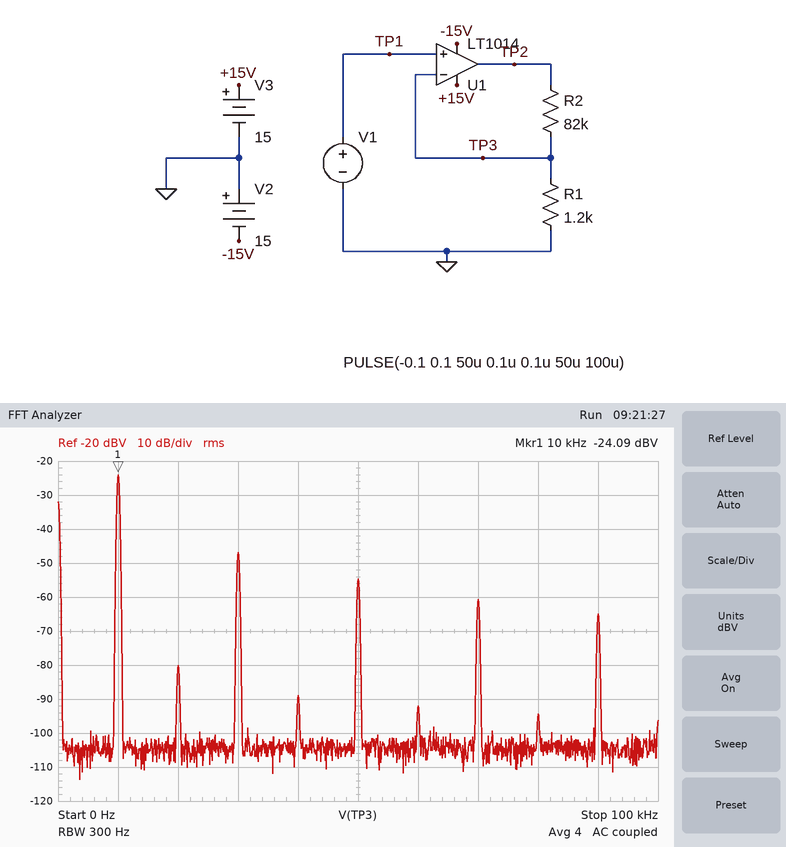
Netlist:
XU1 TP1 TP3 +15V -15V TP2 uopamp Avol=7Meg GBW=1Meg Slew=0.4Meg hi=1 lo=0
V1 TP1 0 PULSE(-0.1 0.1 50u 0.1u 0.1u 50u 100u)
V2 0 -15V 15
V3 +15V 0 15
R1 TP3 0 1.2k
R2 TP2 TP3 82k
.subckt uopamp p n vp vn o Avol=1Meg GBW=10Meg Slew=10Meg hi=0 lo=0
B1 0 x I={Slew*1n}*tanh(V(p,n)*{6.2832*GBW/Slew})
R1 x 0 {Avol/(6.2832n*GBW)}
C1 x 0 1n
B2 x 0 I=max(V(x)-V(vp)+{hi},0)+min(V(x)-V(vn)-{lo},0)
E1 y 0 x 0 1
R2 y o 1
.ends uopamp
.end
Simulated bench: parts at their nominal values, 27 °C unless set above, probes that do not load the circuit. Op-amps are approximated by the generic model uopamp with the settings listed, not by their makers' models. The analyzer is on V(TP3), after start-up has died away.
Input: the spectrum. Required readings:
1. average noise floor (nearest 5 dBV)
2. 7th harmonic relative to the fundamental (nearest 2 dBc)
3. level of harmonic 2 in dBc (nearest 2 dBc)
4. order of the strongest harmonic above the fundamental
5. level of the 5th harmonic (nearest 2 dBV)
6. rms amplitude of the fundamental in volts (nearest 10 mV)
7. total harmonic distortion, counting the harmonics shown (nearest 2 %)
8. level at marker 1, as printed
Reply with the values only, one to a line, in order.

-105 dBV
-36 dBc
-56 dBc
3
-54 dBV
60 mV
8 %
-24.09 dBV
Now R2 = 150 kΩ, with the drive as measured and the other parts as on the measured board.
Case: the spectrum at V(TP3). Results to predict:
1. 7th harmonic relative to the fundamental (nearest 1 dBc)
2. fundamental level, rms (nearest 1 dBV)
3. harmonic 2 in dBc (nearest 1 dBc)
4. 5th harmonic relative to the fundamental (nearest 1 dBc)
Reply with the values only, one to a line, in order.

-35 dBc
-28 dBV
-57 dBc
-29 dBc
